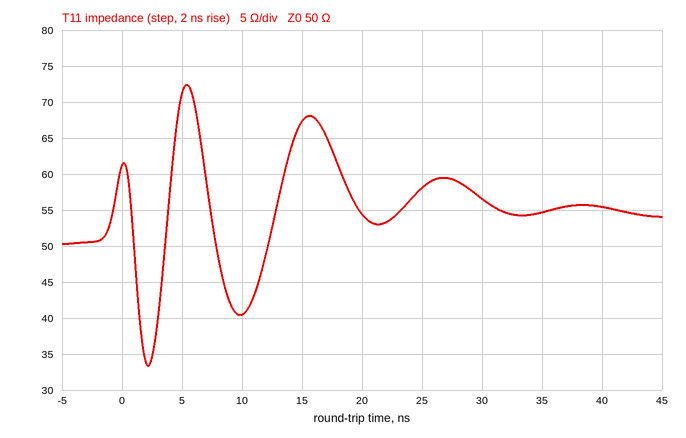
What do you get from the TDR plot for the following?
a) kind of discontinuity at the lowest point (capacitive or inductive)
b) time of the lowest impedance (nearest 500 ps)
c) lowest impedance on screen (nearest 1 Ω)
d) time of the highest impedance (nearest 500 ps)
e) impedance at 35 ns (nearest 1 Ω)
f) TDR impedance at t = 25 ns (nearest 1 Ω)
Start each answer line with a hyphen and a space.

- capacitive
- 2.0 ns
- 33 Ω
- 5.5 ns
- 55 Ω
- 58 Ω
